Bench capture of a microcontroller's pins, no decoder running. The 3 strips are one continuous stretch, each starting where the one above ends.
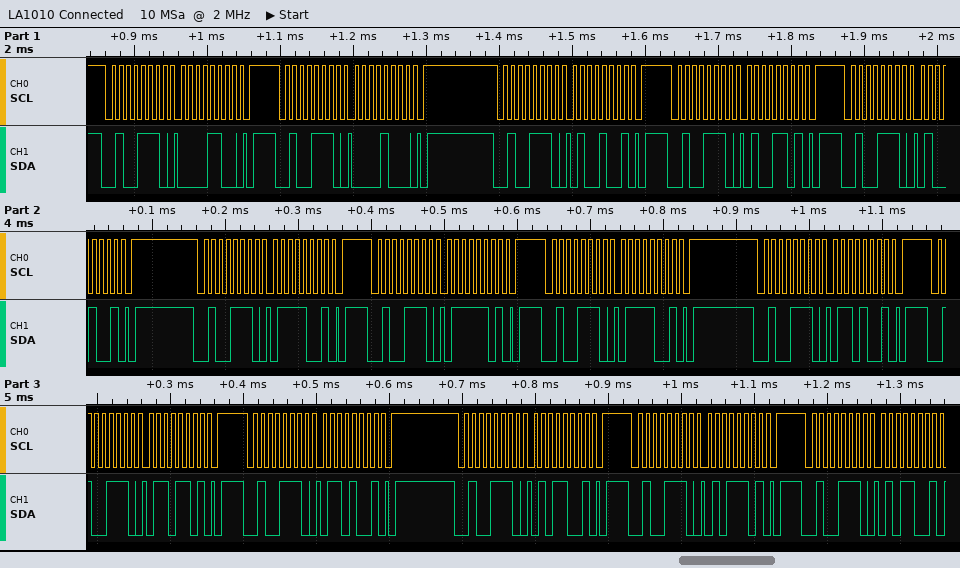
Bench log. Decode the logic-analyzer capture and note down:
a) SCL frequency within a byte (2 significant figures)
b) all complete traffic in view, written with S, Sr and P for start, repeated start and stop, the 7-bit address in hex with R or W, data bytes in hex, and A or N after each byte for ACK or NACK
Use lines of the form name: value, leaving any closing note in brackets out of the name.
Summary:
SCL frequency within a byte: 100 kHz
all complete traffic in view, written with S, Sr and P for start, repeated start and stop, the 7-bit address in hex with R or W, data bytes in hex, and A or N after each byte for ACK or NACK: S 27W A 0C A P S 27W A 08 A P S 27W A 49 A P S 27W A 4D A P S 27W A 49 A P S 27W A 79 A P S 27W A 7D A P S 27W A 79 A P S 27W A 69 A P S 27W A 6D A P S 27W A 69 A P S 27W A 59 A P S 27W A 5D A P S 27W A 59 A
